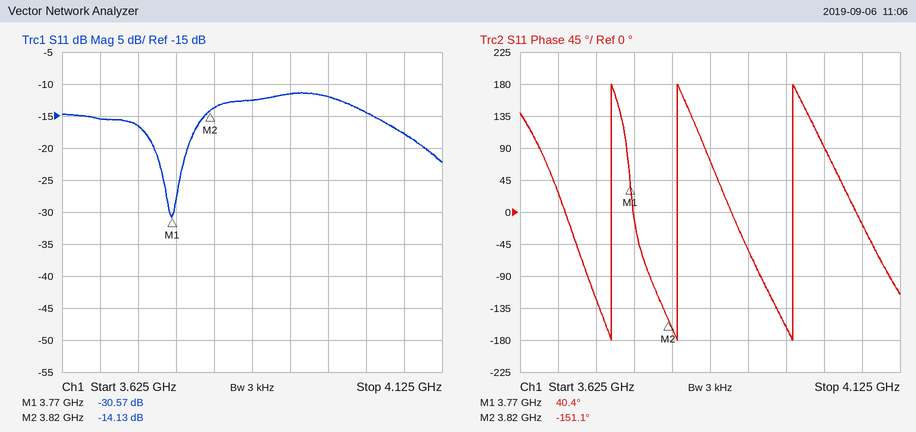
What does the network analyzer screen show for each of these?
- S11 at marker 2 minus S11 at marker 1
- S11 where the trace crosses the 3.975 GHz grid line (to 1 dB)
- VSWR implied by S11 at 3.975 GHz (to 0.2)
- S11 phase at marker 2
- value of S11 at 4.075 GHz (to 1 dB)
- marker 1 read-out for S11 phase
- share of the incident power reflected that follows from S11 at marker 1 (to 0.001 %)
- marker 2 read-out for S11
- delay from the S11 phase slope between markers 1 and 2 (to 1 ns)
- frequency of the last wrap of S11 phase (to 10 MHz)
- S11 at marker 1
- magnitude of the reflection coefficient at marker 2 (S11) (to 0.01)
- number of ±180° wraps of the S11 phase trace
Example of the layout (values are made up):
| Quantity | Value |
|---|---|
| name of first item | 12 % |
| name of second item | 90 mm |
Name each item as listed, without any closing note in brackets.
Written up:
| Quantity | Value |
|---|---|
| S11 at marker 2 minus S11 at marker 1 | 16.44 dB |
| S11 where the trace crosses the 3.975 GHz grid line | -12 dB |
| VSWR implied by S11 at 3.975 GHz | 1.6 |
| S11 phase at marker 2 | -151.1° |
| value of S11 at 4.075 GHz | -18 dB |
| marker 1 read-out for S11 phase | 40.4° |
| share of the incident power reflected that follows from S11 at marker 1 | 0.088 % |
| marker 2 read-out for S11 | -14.13 dB |
| delay from the S11 phase slope between markers 1 and 2 | 11 ns |
| frequency of the last wrap of S11 phase | 3.98 GHz |
| S11 at marker 1 | -30.57 dB |
| magnitude of the reflection coefficient at marker 2 (S11) | 0.20 |
| number of ±180° wraps of the S11 phase trace | 3 |
